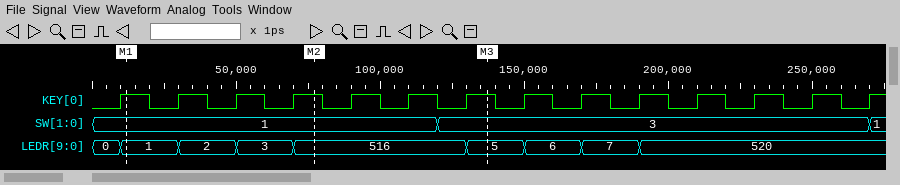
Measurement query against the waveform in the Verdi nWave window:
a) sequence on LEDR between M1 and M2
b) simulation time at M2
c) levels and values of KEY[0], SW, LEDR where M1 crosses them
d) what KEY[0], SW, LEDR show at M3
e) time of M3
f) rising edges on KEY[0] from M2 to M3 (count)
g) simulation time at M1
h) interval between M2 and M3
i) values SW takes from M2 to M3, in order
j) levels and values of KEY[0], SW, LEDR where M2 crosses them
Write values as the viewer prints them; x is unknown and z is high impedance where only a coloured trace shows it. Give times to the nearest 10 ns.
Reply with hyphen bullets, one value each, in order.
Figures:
- 1, 2, 3, 516
- 80 ns
- KEY[0]=1, SW=1, LEDR=1
- KEY[0]=1, SW=3, LEDR=5
- 140 ns
- 3
- 10 ns
- 60 ns
- 1, 3
- KEY[0]=1, SW=1, LEDR=516
